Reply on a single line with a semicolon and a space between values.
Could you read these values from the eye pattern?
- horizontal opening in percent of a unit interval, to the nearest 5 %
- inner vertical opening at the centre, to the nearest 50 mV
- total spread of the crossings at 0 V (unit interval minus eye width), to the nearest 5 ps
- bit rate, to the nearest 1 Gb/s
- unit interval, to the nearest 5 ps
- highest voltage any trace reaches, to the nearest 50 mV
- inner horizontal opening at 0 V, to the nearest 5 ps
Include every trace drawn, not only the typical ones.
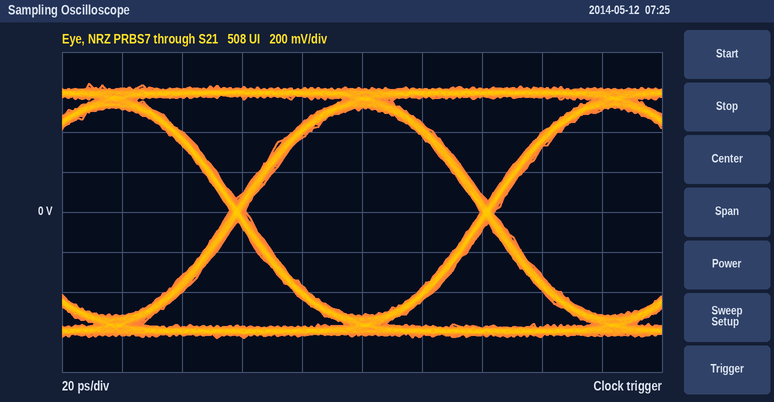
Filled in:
95 %; 1.05 V; 5 ps; 12 Gb/s; 85 ps; 650 mV; 80 ps
